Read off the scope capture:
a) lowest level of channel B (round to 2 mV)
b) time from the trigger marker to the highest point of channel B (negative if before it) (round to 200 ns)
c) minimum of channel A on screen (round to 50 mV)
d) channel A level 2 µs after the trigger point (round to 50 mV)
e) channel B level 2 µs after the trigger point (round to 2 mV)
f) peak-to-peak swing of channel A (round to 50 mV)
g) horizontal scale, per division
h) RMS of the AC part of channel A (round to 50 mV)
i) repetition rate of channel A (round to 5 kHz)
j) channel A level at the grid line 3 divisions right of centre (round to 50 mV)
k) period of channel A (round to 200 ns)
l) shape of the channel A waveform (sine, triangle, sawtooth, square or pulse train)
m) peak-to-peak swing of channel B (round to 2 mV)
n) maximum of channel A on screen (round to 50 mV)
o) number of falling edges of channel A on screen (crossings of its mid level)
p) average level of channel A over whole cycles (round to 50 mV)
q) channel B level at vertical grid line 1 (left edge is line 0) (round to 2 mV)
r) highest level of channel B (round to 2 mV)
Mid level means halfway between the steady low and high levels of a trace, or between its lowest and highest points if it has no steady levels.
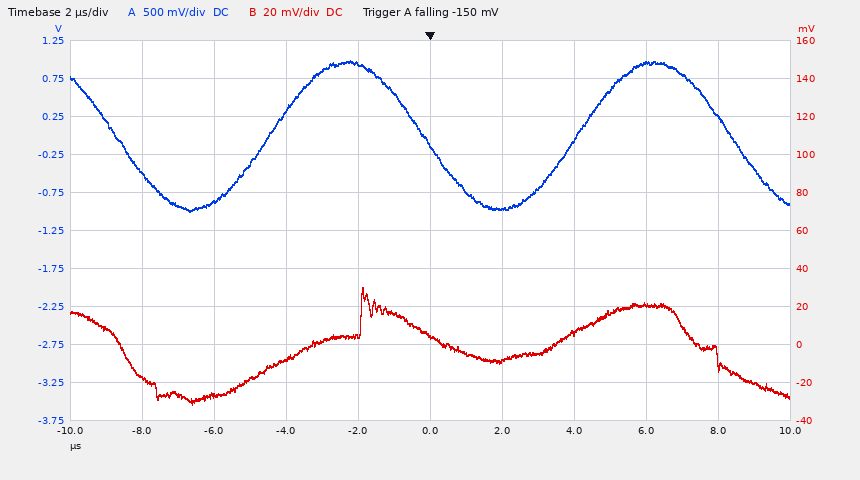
-32 mV
-1.8 µs
-1.00 V
-950 mV
-8 mV
2.00 V
2 µs
700 mV
115 kHz
950 mV
8.6 µs
sine
62 mV
1.00 V
3
0 mV
-18 mV
30 mV
